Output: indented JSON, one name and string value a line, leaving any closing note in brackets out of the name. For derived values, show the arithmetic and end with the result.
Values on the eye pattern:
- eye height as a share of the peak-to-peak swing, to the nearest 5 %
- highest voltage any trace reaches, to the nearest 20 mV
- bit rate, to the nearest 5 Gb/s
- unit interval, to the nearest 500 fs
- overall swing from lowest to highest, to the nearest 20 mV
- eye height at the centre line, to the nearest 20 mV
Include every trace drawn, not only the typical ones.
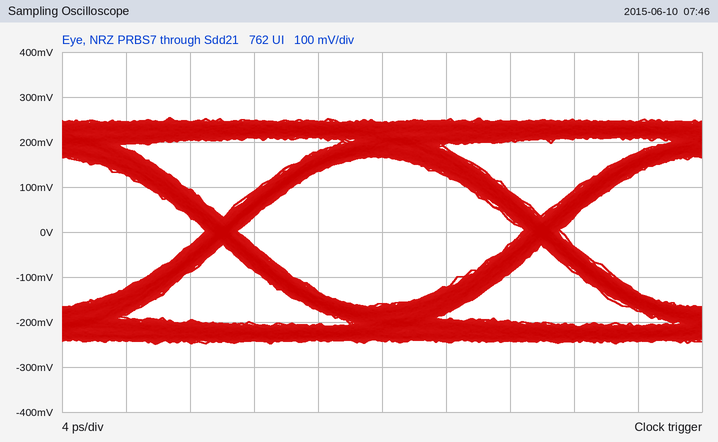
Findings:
{
  "eye height as a share of the peak-to-peak swing, to the nearest 5 %": "320 mV / 500 mV ≈ 64.0 %, so 65 % to the nearest 5 %",
  "highest voltage any trace reaches, to the nearest 20 mV": "260 mV",
  "bit rate, to the nearest 5 Gb/s": "50 Gb/s",
  "unit interval, to the nearest 500 fs": "20.0 ps",
  "overall swing from lowest to highest, to the nearest 20 mV": "500 mV",
  "eye height at the centre line, to the nearest 20 mV": "320 mV"
}
